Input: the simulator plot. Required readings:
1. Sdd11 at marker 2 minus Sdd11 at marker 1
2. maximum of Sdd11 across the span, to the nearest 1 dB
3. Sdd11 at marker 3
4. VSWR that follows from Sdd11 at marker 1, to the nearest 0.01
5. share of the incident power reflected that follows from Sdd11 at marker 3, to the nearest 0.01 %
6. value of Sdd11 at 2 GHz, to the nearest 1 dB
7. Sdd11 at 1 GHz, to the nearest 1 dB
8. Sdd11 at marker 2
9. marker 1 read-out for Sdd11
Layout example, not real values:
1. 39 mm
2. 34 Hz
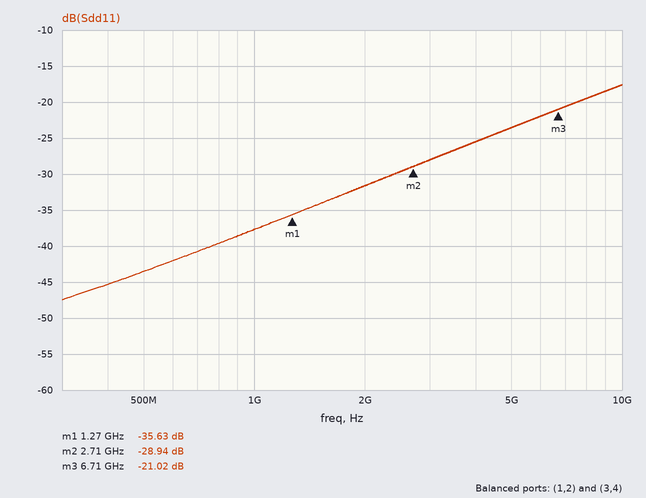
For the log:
1. 6.69 dB
2. -18 dB
3. -21.02 dB
4. 1.03
5. 0.79 %
6. -32 dB
7. -38 dB
8. -28.94 dB
9. -35.63 dB
